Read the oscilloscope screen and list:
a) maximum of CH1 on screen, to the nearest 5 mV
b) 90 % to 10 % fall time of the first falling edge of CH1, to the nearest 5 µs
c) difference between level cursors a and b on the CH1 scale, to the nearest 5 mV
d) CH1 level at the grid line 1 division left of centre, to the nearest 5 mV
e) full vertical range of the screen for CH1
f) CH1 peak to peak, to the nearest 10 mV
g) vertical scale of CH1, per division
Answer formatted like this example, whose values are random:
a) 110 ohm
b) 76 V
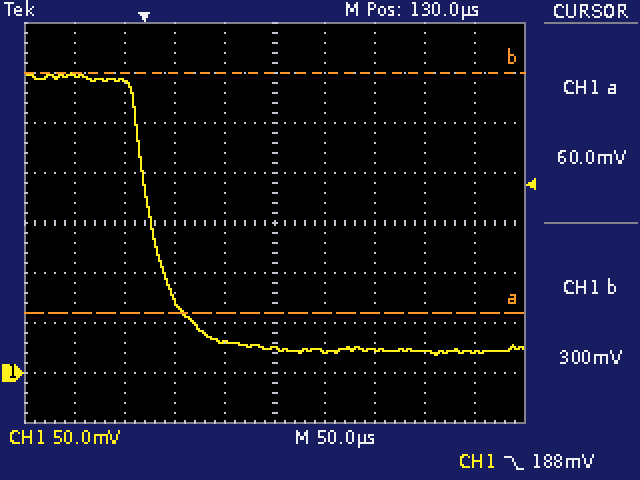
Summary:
a) 300 mV
b) 60 µs
c) 240 mV
d) 30 mV
e) 400 mV
f) 280 mV
g) 50 mV
